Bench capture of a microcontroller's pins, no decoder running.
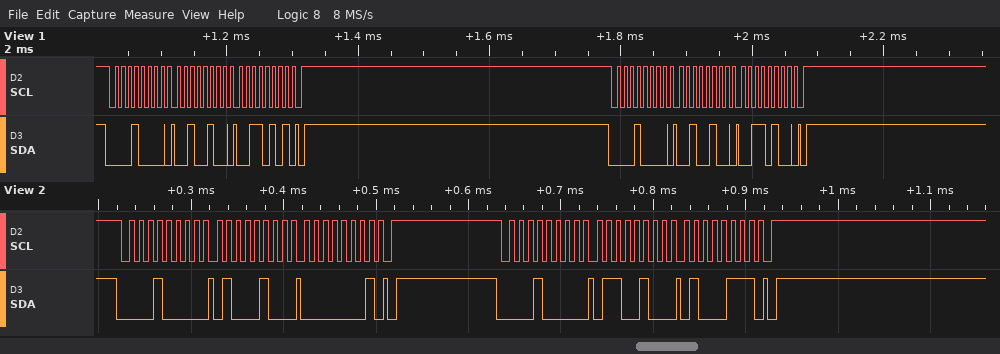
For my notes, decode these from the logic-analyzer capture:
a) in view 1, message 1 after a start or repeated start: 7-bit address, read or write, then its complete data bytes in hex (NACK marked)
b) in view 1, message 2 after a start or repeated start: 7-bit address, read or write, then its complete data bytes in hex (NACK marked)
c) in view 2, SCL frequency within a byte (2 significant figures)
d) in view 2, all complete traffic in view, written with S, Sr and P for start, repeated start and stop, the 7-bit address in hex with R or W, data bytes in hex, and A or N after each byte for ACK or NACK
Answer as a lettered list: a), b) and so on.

a) 0x08 write: 24 35
b) 0x08 write: 24 34
c) 100 kHz
d) S 08W A 44 A 01 A P S 08W A 64 A 47 A P
